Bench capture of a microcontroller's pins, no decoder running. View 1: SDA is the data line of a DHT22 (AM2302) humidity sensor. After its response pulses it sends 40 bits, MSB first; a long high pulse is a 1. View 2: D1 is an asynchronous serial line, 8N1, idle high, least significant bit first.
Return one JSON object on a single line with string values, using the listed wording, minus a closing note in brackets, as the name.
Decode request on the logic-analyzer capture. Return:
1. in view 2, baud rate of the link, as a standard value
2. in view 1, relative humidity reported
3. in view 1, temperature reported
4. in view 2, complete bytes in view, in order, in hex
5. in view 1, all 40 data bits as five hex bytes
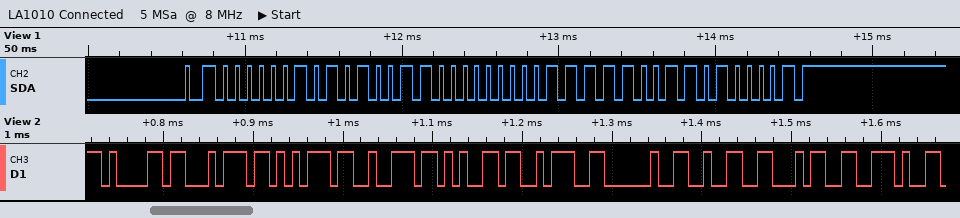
{"in view 2, baud rate of the link, as a standard value": "115200 baud", "in view 1, relative humidity reported": "67.8 %", "in view 1, temperature reported": "24.9 °C", "in view 2, complete bytes in view, in order, in hex": "0x61 0x74 0x75 0x72 0x65 0x3A 0x20 0x32 0x34 0x2E", "in view 1, all 40 data bits as five hex bytes": "02 A6 00 F9 A1"}
